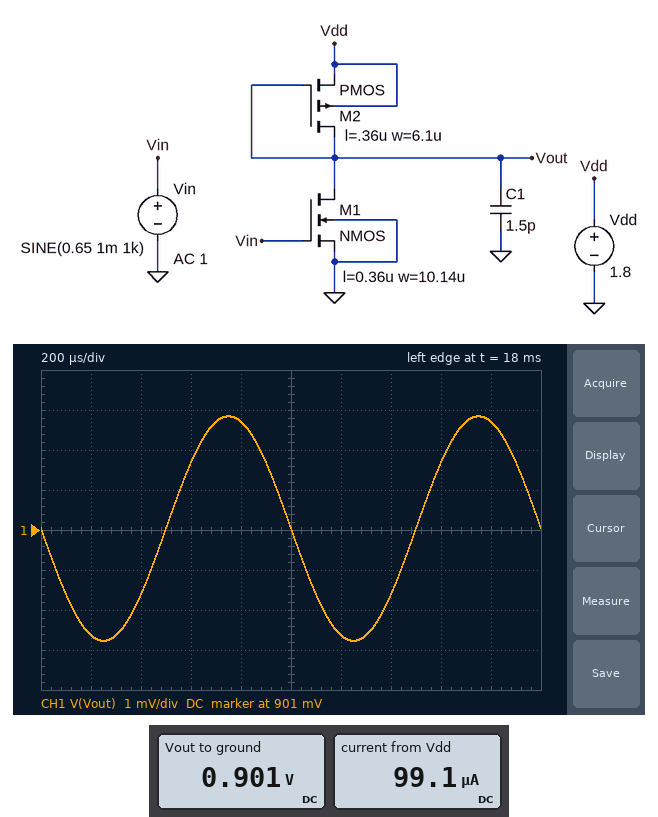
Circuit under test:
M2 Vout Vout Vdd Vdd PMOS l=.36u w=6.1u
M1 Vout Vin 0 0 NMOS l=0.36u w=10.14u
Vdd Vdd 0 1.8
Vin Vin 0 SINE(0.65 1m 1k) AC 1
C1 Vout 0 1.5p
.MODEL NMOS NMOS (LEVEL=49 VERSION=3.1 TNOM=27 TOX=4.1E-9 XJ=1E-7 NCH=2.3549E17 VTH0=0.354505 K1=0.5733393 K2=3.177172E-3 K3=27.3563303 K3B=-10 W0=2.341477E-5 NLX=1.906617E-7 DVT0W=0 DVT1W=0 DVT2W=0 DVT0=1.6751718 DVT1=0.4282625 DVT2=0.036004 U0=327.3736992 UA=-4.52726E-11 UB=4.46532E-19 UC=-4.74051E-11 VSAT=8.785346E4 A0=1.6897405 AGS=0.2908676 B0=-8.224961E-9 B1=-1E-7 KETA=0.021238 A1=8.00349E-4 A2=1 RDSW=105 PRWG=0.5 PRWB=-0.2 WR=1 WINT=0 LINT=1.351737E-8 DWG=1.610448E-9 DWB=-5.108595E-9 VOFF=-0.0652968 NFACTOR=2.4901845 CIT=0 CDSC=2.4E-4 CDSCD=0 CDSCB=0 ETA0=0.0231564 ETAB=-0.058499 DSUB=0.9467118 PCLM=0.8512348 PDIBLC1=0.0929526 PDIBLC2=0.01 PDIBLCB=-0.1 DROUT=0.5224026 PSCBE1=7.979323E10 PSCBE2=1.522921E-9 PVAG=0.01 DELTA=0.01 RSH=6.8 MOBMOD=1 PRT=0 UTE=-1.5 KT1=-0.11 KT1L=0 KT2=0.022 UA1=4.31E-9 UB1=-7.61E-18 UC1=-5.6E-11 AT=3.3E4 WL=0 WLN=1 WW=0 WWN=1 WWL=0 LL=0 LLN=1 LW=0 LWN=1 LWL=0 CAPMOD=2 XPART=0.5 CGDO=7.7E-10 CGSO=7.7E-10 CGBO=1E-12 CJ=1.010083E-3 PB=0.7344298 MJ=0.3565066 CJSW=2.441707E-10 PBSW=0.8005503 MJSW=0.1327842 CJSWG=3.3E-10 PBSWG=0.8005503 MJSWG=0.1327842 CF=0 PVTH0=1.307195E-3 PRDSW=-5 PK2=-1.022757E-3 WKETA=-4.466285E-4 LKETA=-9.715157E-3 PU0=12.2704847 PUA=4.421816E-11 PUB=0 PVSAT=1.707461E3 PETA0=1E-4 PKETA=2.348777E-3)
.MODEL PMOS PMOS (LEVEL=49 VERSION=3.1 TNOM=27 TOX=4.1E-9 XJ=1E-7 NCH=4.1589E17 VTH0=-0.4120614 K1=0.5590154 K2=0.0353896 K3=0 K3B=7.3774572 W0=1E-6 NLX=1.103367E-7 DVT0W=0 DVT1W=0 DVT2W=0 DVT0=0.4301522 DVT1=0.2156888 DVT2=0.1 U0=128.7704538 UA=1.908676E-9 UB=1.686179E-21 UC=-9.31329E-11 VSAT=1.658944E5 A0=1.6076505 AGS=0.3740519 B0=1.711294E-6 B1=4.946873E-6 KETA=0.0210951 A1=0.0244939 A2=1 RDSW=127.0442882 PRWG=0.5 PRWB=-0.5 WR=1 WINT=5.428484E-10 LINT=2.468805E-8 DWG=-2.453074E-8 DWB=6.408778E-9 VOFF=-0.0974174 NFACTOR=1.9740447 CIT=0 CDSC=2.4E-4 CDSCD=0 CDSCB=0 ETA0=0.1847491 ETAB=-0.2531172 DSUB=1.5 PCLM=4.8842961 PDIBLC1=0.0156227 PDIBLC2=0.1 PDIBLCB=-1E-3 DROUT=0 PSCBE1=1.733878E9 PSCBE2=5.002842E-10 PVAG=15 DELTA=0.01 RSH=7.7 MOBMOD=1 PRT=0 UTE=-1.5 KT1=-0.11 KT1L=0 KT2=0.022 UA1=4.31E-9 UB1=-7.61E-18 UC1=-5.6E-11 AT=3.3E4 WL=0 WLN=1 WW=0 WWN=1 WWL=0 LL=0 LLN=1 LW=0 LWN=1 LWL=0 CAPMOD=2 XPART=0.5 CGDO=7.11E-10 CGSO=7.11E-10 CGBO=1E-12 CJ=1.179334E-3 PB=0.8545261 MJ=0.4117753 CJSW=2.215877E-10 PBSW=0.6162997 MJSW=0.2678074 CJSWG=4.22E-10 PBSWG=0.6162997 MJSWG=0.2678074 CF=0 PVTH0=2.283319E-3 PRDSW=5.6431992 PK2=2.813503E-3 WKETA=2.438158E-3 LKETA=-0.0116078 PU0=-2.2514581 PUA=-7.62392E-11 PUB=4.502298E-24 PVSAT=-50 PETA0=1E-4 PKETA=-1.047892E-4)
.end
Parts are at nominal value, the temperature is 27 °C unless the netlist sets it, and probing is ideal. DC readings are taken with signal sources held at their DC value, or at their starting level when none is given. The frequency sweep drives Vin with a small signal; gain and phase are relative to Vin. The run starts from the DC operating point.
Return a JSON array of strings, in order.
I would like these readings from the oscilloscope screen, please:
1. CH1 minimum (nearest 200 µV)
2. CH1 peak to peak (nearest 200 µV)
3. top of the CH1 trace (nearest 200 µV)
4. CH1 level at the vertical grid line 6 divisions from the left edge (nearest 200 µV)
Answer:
["898.2 mV", "5.6 mV", "903.8 mV", "898.4 mV"]
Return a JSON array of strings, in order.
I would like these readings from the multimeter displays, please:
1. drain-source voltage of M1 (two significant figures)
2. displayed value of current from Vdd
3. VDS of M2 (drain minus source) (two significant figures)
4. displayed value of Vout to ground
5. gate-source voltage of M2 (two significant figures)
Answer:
["900 mV", "99.1 µA", "-900 mV", "0.901 V", "-900 mV"]
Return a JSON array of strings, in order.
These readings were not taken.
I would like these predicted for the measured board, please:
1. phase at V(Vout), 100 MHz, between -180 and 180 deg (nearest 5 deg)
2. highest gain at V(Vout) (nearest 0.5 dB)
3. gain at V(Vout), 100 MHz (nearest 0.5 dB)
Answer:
["115 deg", "9.0 dB", "1.0 dB"]
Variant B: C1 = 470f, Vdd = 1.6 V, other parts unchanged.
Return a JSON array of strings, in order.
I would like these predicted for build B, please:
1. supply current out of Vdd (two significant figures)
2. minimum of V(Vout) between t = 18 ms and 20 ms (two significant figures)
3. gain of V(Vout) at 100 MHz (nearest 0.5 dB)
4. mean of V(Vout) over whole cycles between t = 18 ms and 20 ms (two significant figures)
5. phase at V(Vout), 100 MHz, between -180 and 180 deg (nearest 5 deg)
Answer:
["97 µA", "700 mV", "7.0 dB", "710 mV", "145 deg"]
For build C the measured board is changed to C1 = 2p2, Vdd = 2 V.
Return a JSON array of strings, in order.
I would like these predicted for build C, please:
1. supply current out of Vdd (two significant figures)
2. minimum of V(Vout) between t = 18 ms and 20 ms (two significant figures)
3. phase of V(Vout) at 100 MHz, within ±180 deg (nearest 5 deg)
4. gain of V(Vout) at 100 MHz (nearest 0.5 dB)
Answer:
["100 µA", "1.1 V", "105 deg", "-1.5 dB"]
